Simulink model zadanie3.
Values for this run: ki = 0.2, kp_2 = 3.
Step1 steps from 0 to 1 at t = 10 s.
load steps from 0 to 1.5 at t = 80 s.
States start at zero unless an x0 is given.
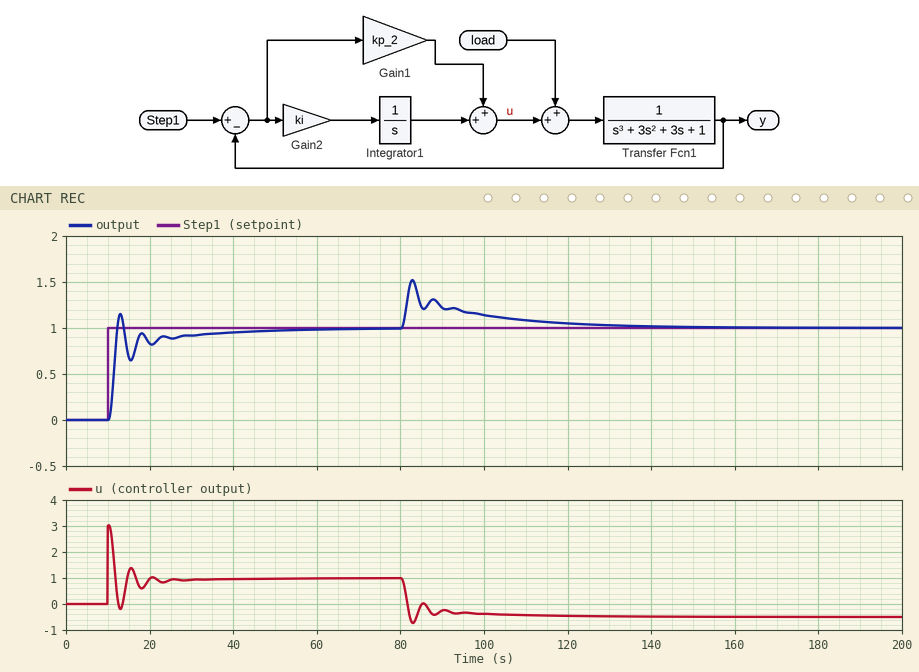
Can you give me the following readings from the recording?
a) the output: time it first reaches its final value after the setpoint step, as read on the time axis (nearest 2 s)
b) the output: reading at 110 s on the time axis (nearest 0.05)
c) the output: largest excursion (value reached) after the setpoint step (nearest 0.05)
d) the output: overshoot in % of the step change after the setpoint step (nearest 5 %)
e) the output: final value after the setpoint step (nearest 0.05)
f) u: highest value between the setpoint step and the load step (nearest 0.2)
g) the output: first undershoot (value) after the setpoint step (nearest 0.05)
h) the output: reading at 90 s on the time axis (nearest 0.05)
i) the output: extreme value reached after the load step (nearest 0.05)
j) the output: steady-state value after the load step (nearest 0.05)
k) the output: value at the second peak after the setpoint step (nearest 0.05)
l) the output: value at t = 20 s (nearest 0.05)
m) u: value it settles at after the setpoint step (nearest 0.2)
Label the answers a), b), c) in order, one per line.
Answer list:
a) 12 s
b) 1.10
c) 1.15
d) 15 %
e) 1.00
f) 3.0
g) 0.65
h) 1.20
i) 1.50
j) 1.00
k) 0.95
l) 0.85
m) 1.0
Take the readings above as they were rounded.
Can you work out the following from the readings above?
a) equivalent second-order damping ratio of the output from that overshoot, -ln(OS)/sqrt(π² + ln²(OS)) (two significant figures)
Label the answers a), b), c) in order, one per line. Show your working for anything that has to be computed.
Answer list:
a) ln(0.15) = -1.897; 1.897 / sqrt(9.870 + 3.599) = 0.52
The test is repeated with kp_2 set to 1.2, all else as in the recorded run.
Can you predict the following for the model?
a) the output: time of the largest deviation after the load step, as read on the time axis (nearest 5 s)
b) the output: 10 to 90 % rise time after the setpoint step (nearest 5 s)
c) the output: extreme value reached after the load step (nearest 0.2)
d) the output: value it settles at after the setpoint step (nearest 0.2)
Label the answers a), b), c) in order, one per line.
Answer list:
a) 85 s
b) 15 s
c) 1.8
d) 1.0
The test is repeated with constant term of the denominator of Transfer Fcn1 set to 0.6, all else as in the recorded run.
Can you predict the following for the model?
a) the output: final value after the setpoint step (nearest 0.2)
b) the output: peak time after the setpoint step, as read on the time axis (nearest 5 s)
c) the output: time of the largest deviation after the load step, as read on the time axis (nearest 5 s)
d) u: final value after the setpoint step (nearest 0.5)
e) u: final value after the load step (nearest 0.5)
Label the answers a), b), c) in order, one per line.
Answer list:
a) 1.0
b) 15 s
c) 85 s
d) 0.5
e) -1.0
